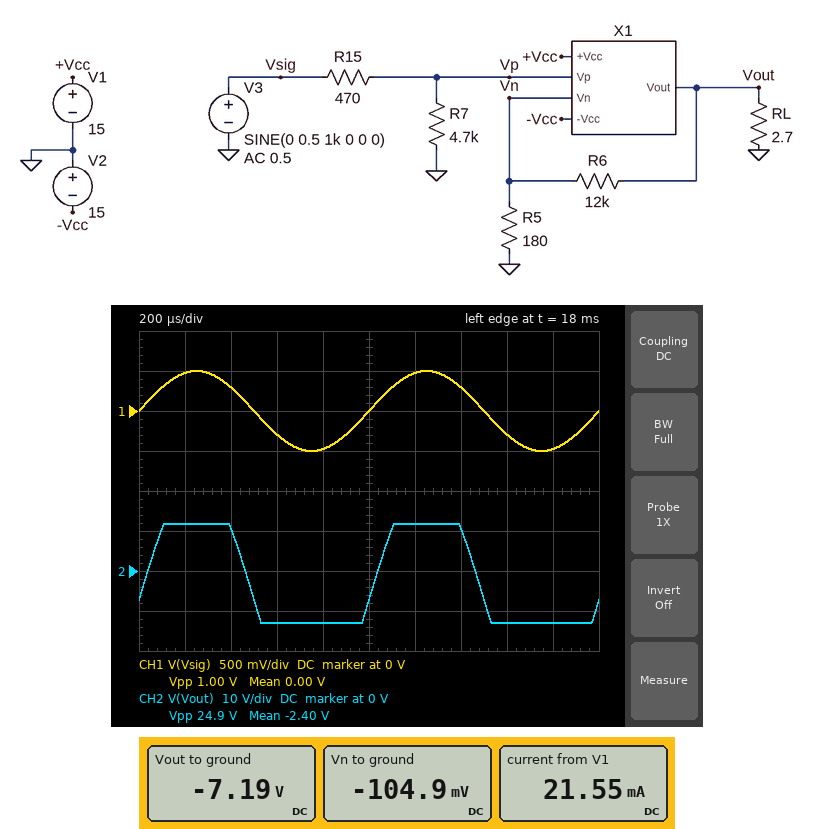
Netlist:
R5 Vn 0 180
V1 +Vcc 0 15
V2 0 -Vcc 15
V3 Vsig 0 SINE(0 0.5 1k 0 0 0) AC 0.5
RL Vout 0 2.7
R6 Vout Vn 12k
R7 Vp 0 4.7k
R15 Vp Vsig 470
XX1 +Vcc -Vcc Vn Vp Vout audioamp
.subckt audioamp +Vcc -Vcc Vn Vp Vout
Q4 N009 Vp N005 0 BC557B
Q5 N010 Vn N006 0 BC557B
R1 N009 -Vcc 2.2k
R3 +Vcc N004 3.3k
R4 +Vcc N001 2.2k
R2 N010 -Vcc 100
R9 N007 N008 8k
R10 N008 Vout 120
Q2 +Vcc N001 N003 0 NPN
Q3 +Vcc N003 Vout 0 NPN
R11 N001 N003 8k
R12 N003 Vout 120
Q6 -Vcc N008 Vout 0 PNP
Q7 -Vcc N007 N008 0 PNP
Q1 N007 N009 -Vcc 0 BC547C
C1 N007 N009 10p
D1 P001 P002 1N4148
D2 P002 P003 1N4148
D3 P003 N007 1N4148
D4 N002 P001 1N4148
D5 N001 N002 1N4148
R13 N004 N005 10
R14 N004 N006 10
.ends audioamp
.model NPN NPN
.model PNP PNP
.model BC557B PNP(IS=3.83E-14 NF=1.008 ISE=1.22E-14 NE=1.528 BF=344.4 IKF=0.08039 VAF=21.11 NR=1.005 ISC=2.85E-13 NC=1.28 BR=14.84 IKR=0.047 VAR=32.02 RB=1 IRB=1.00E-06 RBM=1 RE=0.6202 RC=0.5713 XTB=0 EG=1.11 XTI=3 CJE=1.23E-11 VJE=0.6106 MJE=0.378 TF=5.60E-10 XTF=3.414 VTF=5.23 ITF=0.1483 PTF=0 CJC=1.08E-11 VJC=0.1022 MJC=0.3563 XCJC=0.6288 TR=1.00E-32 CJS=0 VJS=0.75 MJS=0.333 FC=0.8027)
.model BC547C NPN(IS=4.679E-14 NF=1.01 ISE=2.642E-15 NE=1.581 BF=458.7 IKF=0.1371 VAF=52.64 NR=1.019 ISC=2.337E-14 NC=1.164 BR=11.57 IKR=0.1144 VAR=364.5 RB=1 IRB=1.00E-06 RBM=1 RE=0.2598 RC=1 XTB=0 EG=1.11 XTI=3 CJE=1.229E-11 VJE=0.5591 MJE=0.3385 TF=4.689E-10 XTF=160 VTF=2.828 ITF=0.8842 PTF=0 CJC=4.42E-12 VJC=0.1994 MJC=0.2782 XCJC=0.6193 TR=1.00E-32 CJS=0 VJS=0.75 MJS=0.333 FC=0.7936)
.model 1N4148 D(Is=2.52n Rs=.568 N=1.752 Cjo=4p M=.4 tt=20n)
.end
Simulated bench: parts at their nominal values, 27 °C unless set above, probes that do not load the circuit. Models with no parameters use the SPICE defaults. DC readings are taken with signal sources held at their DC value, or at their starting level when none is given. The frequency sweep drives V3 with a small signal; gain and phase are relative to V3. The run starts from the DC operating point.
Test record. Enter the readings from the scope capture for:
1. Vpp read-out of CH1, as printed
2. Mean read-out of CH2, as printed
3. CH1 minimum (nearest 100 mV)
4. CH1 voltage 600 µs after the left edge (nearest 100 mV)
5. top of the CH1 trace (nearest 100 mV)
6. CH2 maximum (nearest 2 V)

1.00 V
-2.40 V
-500 mV
-300 mV
500 mV
12 V
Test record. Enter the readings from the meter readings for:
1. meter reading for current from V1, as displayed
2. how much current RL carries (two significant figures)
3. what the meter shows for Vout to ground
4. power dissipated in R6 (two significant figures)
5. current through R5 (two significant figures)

21.55 mA
2.7 A
-7.19 V
4.2 mW
580 µA
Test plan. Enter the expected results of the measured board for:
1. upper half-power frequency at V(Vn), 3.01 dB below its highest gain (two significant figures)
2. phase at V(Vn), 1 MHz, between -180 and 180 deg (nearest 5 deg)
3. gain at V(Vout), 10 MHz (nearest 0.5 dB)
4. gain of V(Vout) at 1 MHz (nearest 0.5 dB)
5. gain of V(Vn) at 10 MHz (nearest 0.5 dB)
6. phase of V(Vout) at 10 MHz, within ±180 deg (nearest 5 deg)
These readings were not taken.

2.0 MHz
-30 deg
19.0 dB
35.0 dB
-24.5 dB
-130 deg
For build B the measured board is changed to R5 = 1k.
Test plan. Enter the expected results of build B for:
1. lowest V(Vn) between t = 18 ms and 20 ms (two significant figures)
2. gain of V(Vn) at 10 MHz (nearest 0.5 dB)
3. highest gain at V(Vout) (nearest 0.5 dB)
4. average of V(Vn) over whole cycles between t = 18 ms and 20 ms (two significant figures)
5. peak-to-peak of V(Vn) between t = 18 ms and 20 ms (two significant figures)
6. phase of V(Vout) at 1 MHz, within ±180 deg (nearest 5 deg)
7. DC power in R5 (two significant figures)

-560 mV
-8.5 dB
24.0 dB
-110 mV
910 mV
-5 deg
11 µW
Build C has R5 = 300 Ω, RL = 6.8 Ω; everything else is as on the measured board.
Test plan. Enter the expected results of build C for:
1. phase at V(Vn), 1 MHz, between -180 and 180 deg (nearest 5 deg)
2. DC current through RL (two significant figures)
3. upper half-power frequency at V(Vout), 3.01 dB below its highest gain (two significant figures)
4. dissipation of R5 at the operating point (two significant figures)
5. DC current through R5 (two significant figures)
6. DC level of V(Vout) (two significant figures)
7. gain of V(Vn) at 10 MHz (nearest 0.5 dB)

-20 deg
650 mA
3.9 MHz
37 µW
350 µA
-4.4 V
-20.0 dB
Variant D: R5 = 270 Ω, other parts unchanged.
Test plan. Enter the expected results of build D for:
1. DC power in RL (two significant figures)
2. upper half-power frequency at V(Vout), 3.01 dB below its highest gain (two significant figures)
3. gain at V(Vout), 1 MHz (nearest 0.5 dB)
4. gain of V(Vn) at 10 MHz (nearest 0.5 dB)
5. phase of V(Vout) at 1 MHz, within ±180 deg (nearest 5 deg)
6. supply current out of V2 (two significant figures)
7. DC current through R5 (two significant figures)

8.8 W
3.5 MHz
32.0 dB
-21.0 dB
-20 deg
1.8 A
390 µA
